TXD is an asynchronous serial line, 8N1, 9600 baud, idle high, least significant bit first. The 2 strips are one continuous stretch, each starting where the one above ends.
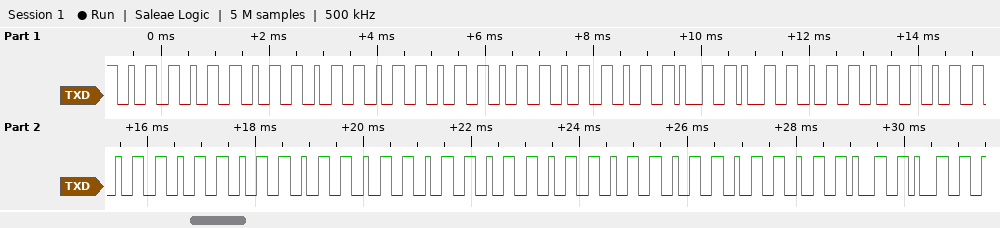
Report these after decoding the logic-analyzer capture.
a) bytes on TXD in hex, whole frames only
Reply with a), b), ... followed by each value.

a) 32 32 32 32 32 32 32 32 32 31 31 32 32 32 32 32 32 32 32 32 32 32 32 32 32 32 31 31
